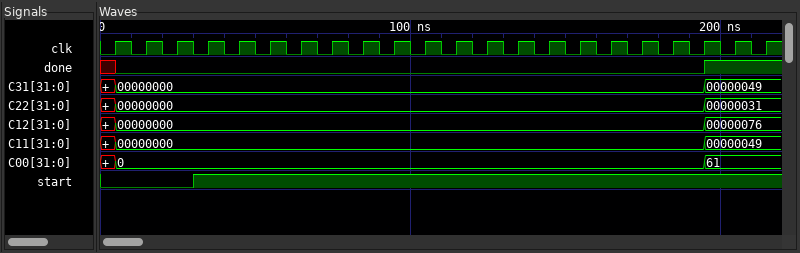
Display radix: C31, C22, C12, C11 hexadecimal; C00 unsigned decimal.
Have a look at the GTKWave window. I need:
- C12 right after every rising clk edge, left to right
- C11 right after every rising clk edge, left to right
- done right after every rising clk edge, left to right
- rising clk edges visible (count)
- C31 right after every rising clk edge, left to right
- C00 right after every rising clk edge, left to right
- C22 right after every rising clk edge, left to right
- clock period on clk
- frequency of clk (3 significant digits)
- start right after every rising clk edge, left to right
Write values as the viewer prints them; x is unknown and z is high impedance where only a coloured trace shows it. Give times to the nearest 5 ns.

00000000, 00000000, 00000000, 00000000, 00000000, 00000000, 00000000, 00000000, 00000000, 00000000, 00000000, 00000000, 00000000, 00000000, 00000000, 00000000, 00000000, 00000000, 00000000, 00000076, 00000076, 00000076
00000000, 00000000, 00000000, 00000000, 00000000, 00000000, 00000000, 00000000, 00000000, 00000000, 00000000, 00000000, 00000000, 00000000, 00000000, 00000000, 00000000, 00000000, 00000000, 00000049, 00000049, 00000049
0 0 0 0 0 0 0 0 0 0 0 0 0 0 0 0 0 0 0 1 1 1
22
00000000, 00000000, 00000000, 00000000, 00000000, 00000000, 00000000, 00000000, 00000000, 00000000, 00000000, 00000000, 00000000, 00000000, 00000000, 00000000, 00000000, 00000000, 00000000, 00000049, 00000049, 00000049
0, 0, 0, 0, 0, 0, 0, 0, 0, 0, 0, 0, 0, 0, 0, 0, 0, 0, 0, 61, 61, 61
00000000, 00000000, 00000000, 00000000, 00000000, 00000000, 00000000, 00000000, 00000000, 00000000, 00000000, 00000000, 00000000, 00000000, 00000000, 00000000, 00000000, 00000000, 00000000, 00000031, 00000031, 00000031
10 ns
100 MHz
0 0 0 1 1 1 1 1 1 1 1 1 1 1 1 1 1 1 1 1 1 1
